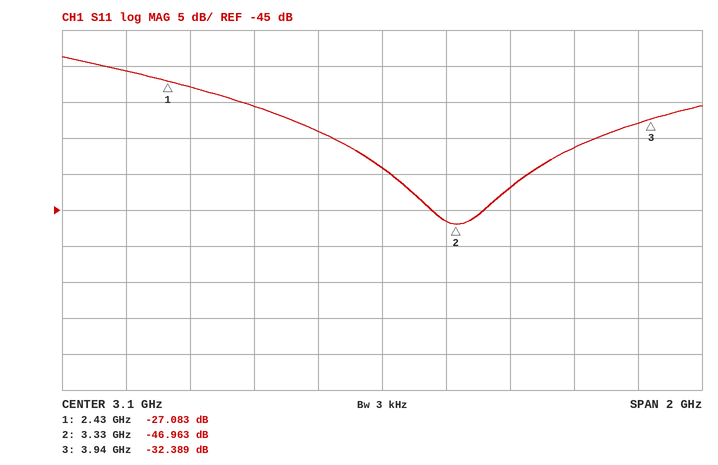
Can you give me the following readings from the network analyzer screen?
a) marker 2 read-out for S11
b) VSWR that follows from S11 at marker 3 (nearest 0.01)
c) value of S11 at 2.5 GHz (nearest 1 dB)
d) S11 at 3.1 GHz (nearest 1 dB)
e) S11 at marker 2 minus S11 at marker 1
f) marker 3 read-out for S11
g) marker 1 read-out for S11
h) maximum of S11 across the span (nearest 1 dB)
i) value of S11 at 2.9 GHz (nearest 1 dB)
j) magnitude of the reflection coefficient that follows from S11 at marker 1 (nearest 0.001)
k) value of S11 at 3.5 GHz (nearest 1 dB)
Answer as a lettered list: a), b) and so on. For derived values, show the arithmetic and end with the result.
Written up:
a) -46.963 dB
b) (1 + 0.0240)/(1 − 0.0240) ≈ 1.05
c) -28 dB
d) -39 dB
e) -46.963 − (-27.083) = -19.880 dB
f) -32.389 dB
g) -27.083 dB
h) -24 dB
i) -34 dB
j) 10^(-27.083/20) ≈ 0.044
k) -42 dB
